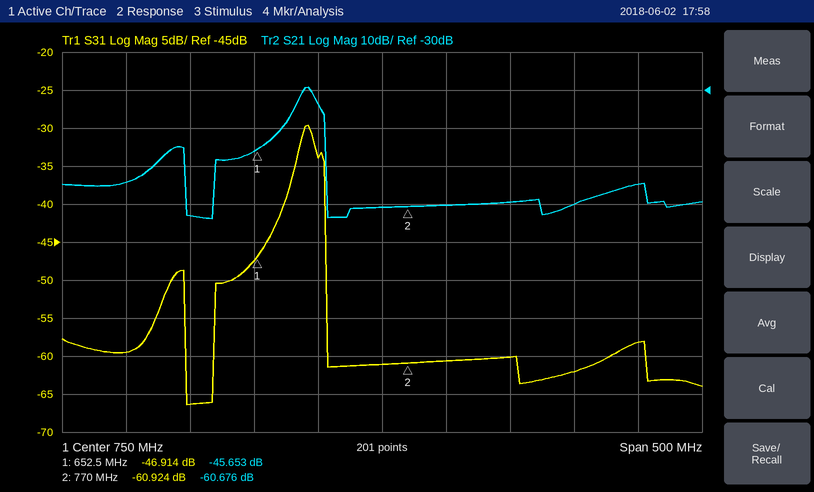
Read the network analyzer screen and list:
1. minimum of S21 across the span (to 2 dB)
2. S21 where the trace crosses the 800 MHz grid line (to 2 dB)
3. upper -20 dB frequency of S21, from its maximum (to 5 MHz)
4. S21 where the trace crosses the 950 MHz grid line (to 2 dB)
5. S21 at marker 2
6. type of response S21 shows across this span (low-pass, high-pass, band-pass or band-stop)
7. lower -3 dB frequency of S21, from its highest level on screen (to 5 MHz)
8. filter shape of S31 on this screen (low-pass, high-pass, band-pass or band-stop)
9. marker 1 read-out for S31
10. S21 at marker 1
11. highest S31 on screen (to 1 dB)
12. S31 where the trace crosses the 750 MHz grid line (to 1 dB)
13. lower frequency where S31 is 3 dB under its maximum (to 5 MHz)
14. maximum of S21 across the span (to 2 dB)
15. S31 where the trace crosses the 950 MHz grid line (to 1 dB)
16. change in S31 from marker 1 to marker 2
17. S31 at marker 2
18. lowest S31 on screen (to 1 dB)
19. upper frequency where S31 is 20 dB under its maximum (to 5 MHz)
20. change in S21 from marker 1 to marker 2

-64 dB
-60 dB
705 MHz
-54 dB
-60.676 dB
band-pass
685 MHz
band-pass
-46.914 dB
-45.653 dB
-30 dB
-61 dB
685 MHz
-30 dB
-58 dB
-14.010 dB
-60.924 dB
-66 dB
705 MHz
-15.023 dB
